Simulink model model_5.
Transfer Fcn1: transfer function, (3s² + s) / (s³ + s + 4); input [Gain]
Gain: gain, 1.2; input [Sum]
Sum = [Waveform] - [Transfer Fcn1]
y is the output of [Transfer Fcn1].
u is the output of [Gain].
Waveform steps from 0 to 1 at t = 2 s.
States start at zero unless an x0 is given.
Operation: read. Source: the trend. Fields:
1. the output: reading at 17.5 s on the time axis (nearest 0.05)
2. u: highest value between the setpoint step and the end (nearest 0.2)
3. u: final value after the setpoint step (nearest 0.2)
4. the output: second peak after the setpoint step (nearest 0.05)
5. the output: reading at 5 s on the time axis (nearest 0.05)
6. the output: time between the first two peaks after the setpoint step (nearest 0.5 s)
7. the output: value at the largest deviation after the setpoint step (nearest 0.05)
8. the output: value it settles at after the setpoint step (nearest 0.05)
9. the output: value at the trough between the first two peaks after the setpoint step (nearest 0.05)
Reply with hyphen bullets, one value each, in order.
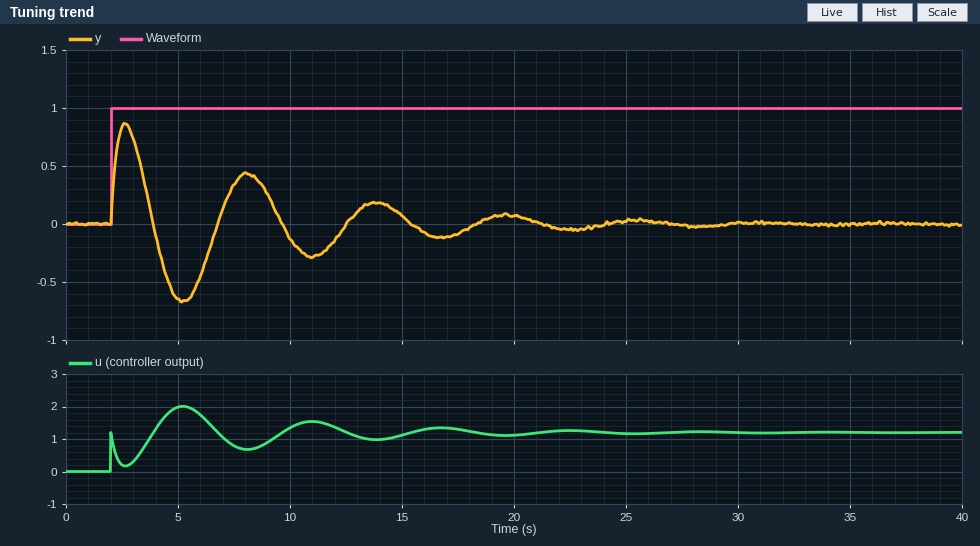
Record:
- -0.10
- 2.0
- 1.2
- 0.45
- -0.65
- 5.5 s
- 0.85
- 0.00
- -0.65
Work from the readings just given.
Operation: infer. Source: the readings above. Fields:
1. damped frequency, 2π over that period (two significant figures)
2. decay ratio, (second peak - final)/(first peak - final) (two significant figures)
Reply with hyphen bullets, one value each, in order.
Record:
- 1.1 rad/s
- 0.53
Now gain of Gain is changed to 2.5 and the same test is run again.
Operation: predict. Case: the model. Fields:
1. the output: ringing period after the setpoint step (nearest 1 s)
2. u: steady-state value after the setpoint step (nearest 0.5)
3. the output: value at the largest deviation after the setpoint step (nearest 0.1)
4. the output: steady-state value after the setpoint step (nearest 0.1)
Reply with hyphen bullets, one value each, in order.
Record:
- 8 s
- 2.5
- 1.0
- 0.0
